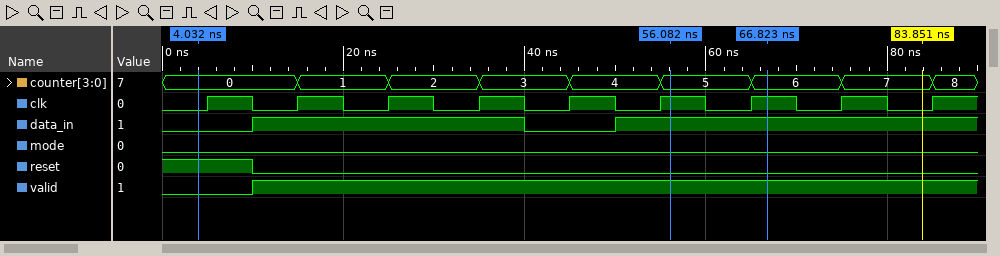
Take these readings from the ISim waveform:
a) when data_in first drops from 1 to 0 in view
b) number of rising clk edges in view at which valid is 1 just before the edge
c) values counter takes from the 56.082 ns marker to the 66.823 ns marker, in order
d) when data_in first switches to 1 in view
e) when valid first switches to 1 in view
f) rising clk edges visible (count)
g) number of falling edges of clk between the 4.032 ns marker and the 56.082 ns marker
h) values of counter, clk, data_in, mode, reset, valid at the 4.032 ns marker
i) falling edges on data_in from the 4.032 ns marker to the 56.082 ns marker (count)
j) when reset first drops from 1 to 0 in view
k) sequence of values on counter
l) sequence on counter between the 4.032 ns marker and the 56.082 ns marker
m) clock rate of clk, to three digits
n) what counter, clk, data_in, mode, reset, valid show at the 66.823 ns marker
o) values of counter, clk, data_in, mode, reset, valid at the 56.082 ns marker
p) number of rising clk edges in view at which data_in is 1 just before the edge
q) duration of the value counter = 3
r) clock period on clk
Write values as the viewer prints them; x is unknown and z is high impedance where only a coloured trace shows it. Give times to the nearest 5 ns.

40 ns
8
5, 6
10 ns
10 ns
9
5
counter=0, clk=0, data_in=0, mode=0, reset=1, valid=0
1
10 ns
0, 1, 2, 3, 4, 5, 6, 7, 8
0, 1, 2, 3, 4, 5
100 MHz
counter=6, clk=1, data_in=1, mode=0, reset=0, valid=1
counter=5, clk=1, data_in=1, mode=0, reset=0, valid=1
7
10 ns
10 ns
